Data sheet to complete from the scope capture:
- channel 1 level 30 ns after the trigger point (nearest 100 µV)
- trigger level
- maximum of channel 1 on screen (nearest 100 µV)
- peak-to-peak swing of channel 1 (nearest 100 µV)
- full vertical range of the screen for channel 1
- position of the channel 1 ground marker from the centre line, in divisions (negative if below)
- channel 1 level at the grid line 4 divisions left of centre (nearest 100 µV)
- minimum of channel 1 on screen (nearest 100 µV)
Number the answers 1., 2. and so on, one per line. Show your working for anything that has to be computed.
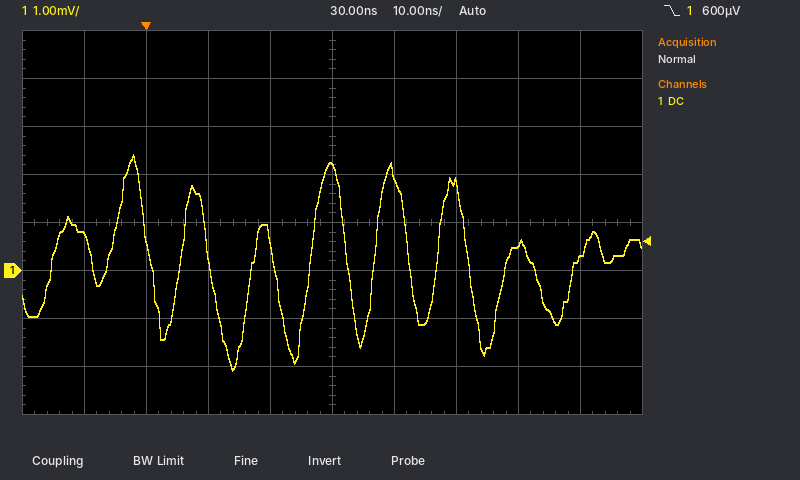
1. 2.2 mV
2. 600 µV
3. 2.4 mV
4. 2.4 mV − (-2.1 mV) = 4.5 mV
5. 8 mV
6. -1.0 div
7. 700 µV
8. -2.1 mV
